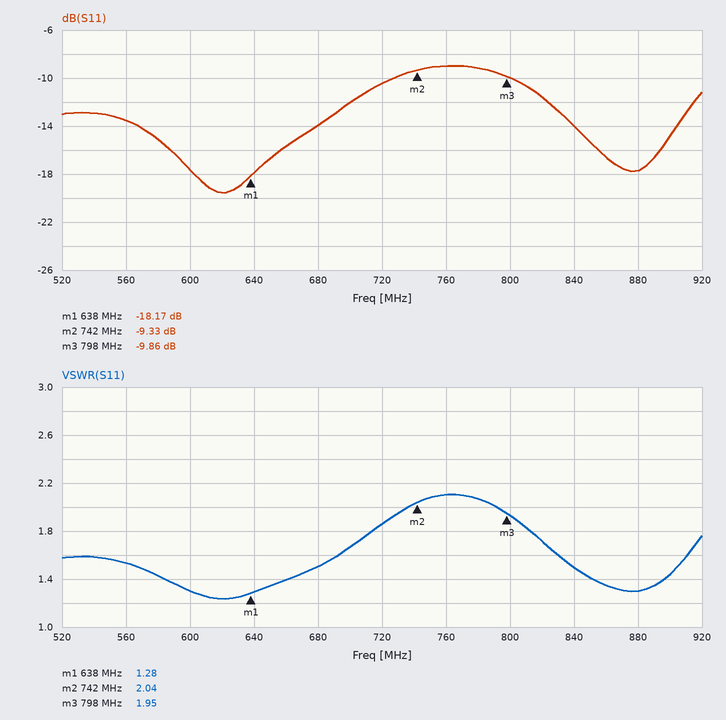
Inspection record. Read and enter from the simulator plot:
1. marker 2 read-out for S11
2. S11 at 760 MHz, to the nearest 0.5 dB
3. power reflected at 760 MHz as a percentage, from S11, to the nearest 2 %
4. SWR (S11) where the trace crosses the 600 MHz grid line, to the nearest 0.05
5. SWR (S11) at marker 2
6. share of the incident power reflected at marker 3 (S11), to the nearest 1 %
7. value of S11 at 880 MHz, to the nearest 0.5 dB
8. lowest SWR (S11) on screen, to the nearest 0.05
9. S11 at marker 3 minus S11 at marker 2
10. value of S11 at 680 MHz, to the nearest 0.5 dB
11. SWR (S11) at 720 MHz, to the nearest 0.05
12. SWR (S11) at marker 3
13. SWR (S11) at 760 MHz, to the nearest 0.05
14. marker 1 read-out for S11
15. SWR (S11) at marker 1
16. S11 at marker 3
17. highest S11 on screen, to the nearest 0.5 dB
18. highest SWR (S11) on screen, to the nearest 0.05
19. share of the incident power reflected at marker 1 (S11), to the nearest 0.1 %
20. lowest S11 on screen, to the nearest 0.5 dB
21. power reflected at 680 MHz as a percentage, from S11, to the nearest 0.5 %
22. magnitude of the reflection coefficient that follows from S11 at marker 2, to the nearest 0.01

-9.33 dB
-9.0 dB
12 %
1.30
2.04
10 %
-17.5 dB
1.25
-0.53 dB
-14.0 dB
1.85
1.95
2.10
-18.17 dB
1.28
-9.86 dB
-9.0 dB
2.10
1.5 %
-19.5 dB
4.0 %
0.34
